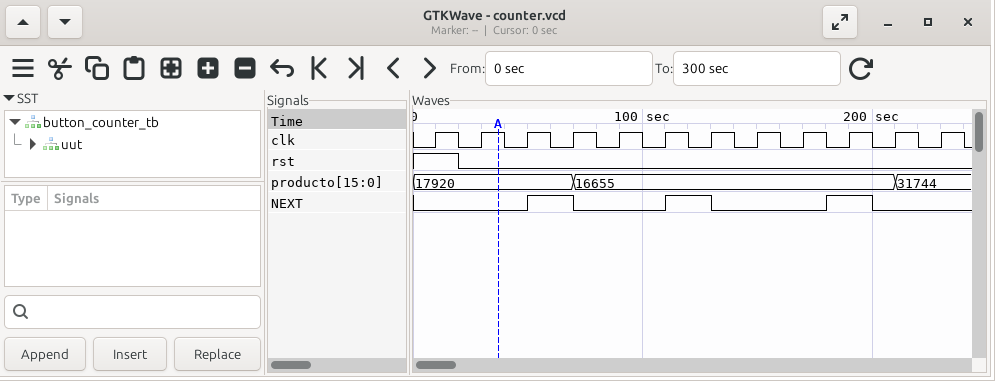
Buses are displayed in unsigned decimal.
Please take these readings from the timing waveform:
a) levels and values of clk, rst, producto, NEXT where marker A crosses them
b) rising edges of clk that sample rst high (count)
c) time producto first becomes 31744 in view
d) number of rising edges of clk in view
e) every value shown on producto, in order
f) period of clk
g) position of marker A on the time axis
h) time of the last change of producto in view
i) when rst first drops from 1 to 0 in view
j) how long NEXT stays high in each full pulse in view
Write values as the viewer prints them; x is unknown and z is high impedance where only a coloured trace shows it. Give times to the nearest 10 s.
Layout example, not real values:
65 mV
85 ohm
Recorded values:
clk=1, rst=0, producto=17920, NEXT=0
1
210 s
12
17920, 16655, 31744
20 s
40 s
210 s
20 s
20 s, 20 s, 20 s
